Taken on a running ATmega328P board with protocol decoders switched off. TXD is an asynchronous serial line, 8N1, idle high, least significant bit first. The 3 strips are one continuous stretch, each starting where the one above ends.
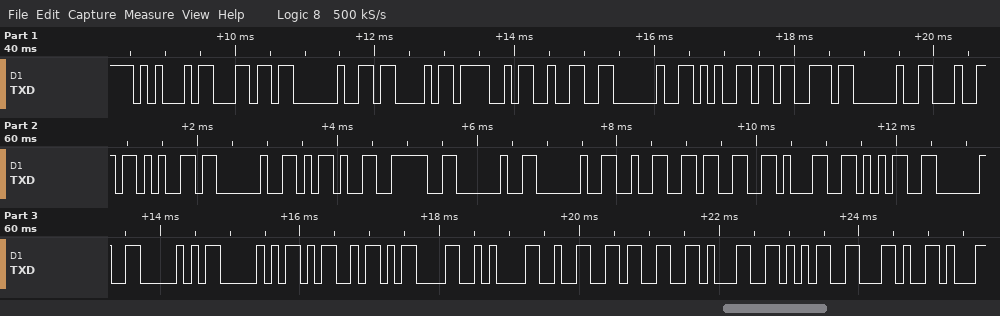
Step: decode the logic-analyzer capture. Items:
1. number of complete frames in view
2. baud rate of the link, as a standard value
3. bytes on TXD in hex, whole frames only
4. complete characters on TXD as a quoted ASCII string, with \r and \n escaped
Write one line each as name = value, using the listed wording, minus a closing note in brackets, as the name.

number of complete frames in view = 32
baud rate of the link, as a standard value = 9600 baud
bytes on TXD in hex, whole frames only = 45 6C 20 43 4F 32 20 65 73 20 64 65 20 2D 3E 20 20 32 33 31 35 20 50 50 4D 0D 0A 32 33 31 35 2C
complete characters on TXD as a quoted ASCII string, with \r and \n escaped = "El CO2 es de ->  2315 PPM\r\n2315,"
